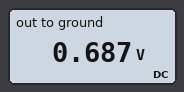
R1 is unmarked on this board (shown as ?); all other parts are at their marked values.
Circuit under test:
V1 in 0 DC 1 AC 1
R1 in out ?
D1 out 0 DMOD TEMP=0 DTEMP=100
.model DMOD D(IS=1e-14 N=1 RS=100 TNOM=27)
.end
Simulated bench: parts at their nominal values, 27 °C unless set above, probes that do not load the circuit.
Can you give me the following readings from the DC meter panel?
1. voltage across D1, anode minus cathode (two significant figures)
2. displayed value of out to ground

690 mV
0.687 V
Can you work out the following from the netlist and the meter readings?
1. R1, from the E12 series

1.5 kΩ
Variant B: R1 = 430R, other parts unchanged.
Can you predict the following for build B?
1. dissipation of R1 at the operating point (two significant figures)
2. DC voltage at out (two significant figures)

150 µW
750 mV
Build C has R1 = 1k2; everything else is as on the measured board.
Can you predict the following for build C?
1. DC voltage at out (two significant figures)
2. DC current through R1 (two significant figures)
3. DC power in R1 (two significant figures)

700 mV
250 µA
77 µW
